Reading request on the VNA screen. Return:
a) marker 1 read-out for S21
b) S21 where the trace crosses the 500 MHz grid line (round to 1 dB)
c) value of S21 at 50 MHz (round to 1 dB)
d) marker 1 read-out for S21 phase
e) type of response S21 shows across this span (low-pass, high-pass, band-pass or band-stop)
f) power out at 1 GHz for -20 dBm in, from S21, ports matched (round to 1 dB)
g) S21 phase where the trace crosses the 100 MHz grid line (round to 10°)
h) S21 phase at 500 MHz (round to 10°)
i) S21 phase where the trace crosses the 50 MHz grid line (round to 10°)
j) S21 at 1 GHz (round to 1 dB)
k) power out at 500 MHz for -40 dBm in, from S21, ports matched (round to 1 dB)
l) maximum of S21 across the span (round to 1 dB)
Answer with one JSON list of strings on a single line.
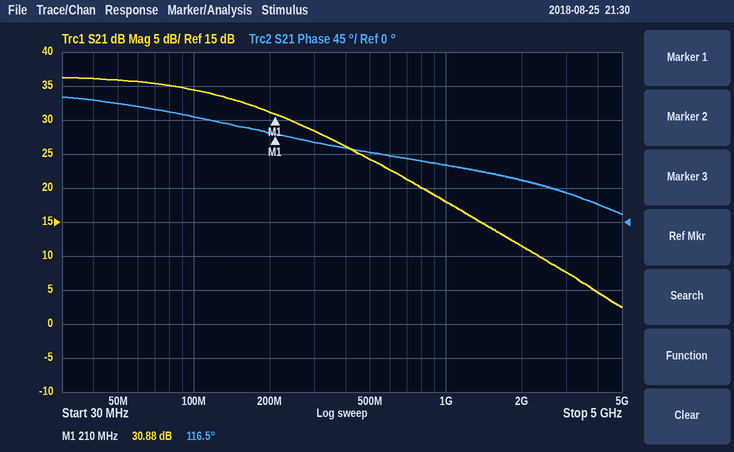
["30.88 dB", "24 dB", "36 dB", "116.5°", "low-pass", "-2 dBm", "140°", "90°", "160°", "18 dB", "-16 dBm", "36 dB"]
